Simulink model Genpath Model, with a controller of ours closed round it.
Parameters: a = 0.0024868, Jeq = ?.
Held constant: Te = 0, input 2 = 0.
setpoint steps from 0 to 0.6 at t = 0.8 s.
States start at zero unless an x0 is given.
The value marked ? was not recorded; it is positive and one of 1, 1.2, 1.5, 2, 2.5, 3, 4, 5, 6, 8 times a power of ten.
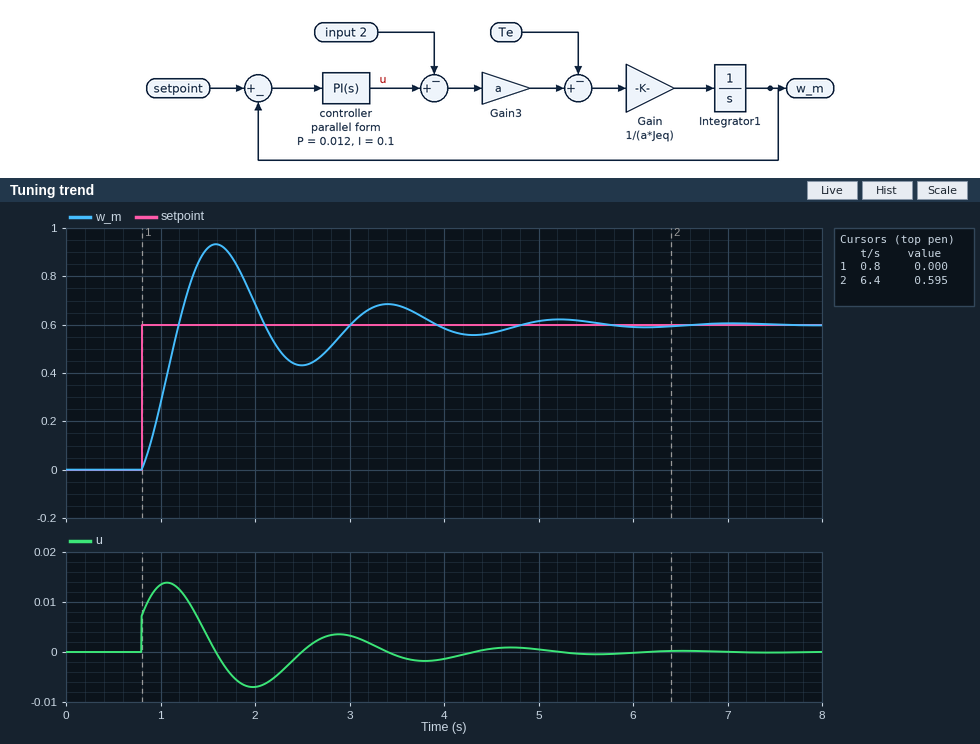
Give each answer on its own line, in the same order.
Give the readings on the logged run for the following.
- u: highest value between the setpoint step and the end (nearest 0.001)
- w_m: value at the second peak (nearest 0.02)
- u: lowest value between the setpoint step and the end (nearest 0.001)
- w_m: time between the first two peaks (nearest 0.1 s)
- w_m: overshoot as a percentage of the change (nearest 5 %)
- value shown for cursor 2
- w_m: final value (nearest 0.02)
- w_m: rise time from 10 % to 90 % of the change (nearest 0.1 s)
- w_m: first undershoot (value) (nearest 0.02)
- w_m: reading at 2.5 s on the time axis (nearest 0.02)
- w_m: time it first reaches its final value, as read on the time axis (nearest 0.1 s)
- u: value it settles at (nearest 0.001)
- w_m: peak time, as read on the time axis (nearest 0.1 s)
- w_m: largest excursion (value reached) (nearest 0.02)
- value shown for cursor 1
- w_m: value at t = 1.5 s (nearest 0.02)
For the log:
0.014
0.68
-0.007
1.8 s
55 %
0.595
0.60
0.3 s
0.44
0.44
1.2 s
0.000
1.6 s
0.94
0.000
0.92
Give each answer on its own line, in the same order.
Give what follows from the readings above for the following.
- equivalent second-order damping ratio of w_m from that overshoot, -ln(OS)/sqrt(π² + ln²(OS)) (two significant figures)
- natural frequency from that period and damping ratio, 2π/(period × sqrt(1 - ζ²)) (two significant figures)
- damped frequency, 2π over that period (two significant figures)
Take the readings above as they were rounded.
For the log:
0.19
3.6 rad/s
3.5 rad/s
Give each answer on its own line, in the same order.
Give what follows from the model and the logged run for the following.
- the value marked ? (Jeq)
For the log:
0.008
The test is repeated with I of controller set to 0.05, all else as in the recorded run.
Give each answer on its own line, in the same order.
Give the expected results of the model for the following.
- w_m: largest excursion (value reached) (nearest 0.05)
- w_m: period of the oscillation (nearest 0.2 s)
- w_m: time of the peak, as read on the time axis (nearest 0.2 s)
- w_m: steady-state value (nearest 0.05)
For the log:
0.85
2.6 s
1.8 s
0.60
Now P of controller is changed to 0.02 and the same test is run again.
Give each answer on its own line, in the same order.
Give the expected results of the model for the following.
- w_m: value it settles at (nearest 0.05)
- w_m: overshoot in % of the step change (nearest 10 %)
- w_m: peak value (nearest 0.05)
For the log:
0.60
40 %
0.85
